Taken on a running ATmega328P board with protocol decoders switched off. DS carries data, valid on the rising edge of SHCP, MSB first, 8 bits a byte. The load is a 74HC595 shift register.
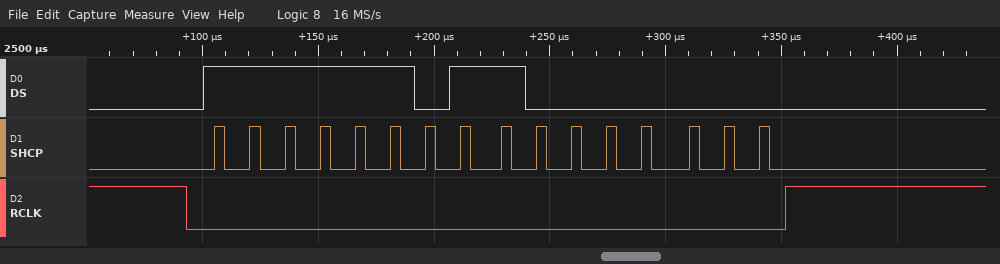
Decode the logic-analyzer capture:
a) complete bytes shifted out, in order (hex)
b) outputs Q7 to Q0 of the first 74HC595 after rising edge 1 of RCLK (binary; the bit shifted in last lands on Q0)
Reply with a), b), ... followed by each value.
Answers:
a) FD 80
b) 10000000
